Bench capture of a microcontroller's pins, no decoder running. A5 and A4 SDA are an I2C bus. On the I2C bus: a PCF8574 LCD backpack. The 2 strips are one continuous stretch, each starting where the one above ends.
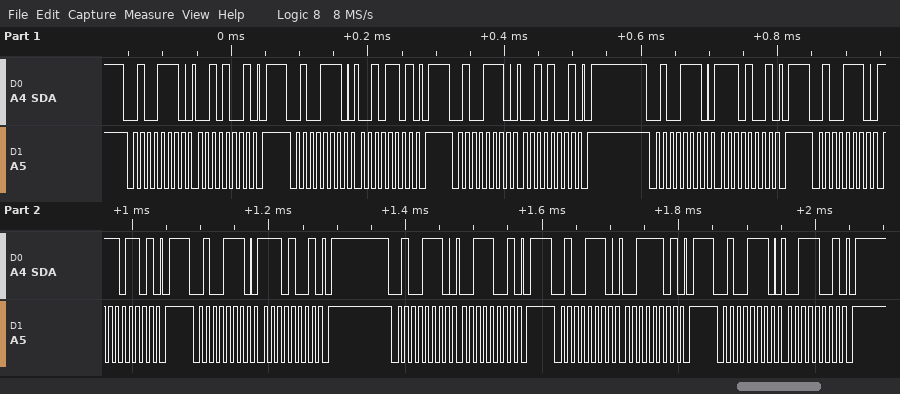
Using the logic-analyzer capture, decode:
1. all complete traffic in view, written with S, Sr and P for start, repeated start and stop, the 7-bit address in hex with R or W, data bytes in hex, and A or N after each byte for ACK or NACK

S 27W A 29 A P S 27W A 2D A P S 27W A 29 A P S 27W A E9 A P S 27W A ED A P S 27W A E9 A P S 27W A 39 A P S 27W A 3D A P S 27W A 39 A P
